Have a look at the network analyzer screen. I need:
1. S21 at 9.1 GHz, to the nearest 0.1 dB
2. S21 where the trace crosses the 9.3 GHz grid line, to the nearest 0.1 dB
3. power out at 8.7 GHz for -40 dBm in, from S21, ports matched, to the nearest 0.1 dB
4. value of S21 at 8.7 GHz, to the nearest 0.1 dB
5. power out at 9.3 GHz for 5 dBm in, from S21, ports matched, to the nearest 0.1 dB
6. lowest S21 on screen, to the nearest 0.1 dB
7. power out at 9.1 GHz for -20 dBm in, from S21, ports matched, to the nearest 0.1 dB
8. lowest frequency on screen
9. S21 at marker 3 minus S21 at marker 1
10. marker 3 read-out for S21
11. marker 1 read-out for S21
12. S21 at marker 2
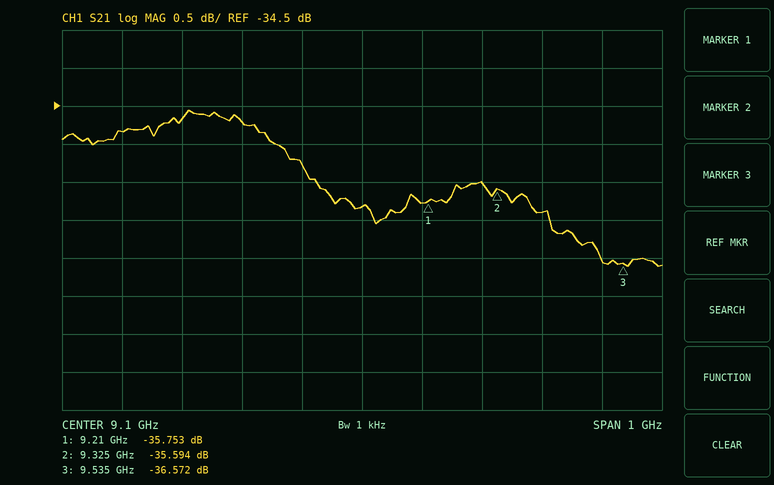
-35.8 dB
-35.5 dB
-74.8 dBm
-34.8 dB
-30.5 dBm
-36.6 dB
-55.8 dBm
8.6 GHz
-0.819 dB
-36.572 dB
-35.753 dB
-35.594 dB
